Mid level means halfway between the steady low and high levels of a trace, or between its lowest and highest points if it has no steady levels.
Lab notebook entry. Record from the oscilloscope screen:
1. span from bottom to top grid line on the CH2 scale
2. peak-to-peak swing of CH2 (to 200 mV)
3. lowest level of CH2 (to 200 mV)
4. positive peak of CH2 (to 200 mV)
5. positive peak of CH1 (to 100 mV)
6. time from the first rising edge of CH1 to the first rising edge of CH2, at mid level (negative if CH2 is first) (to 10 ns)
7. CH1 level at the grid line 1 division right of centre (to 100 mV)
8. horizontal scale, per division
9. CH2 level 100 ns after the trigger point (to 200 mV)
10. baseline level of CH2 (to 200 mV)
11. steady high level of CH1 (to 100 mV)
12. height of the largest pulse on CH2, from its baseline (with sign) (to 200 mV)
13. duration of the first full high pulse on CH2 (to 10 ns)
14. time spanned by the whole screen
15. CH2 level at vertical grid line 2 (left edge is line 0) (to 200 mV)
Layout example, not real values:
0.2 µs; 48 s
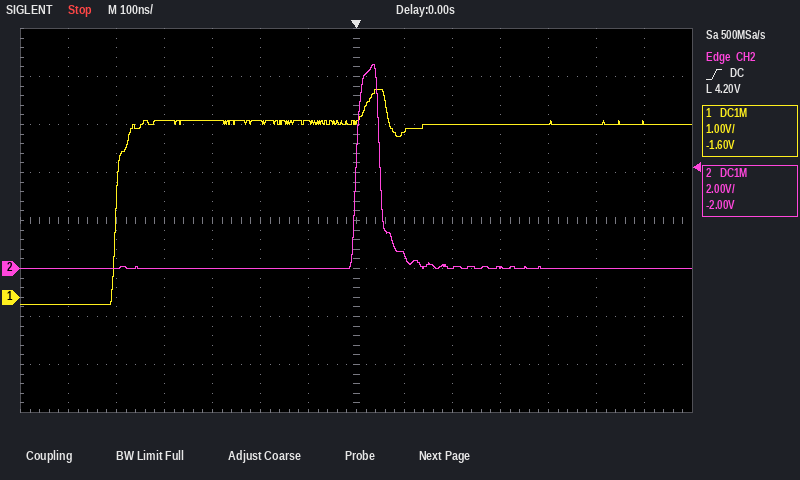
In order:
16 V; 8.4 V; 0.0 V; 8.4 V; 4.3 V; +500 ns; 3.5 V; 100 ns; 600 mV; 0.0 V; 3.6 V; +8.4 V; 50 ns; 1.4 µs; 0.0 V
